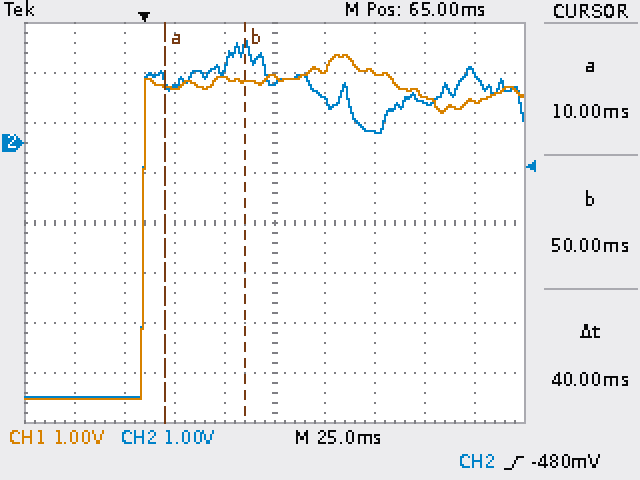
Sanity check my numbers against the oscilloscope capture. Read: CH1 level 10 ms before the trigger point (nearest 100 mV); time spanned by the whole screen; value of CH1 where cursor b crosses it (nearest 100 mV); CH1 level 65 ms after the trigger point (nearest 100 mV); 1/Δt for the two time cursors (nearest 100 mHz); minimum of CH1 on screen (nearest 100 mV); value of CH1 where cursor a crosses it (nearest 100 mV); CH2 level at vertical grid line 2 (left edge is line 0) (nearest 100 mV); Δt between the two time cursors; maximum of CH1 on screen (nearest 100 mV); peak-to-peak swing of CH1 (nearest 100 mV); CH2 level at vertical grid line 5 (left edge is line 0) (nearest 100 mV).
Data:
-5.1 V
250 ms
1.2 V
1.3 V
25.0 Hz
-5.1 V
1.1 V
-5.1 V
40 ms
1.8 V
6.9 V
1.2 V
